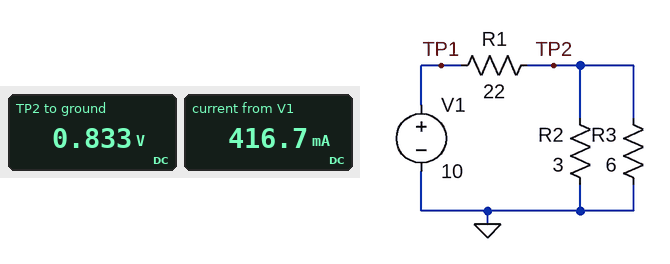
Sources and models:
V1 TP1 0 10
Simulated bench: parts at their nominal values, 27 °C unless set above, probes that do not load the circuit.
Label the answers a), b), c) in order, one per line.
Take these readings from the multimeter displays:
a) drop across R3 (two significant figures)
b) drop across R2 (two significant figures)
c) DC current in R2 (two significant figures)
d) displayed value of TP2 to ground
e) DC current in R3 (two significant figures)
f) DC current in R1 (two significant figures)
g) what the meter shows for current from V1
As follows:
a) 830 mV
b) 830 mV
c) 280 mA
d) 0.833 V
e) 140 mA
f) 420 mA
g) 416.7 mA
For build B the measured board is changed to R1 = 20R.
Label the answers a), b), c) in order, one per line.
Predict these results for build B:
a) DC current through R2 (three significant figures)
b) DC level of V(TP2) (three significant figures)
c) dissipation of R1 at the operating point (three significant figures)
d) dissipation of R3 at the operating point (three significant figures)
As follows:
a) 303 mA
b) 909 mV
c) 4.13 W
d) 138 mW
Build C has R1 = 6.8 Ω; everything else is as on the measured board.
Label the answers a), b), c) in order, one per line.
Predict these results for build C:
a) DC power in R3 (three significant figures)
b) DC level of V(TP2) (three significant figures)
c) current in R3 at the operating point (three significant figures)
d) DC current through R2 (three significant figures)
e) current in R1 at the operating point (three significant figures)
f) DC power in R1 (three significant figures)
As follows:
a) 861 mW
b) 2.27 V
c) 379 mA
d) 758 mA
e) 1.14 A
f) 8.78 W
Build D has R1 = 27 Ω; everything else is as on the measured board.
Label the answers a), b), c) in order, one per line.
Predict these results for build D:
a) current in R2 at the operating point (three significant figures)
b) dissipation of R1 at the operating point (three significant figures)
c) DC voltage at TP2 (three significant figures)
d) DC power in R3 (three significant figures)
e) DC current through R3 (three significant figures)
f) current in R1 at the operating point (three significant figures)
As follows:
a) 230 mA
b) 3.21 W
c) 690 mV
d) 79.3 mW
e) 115 mA
f) 345 mA
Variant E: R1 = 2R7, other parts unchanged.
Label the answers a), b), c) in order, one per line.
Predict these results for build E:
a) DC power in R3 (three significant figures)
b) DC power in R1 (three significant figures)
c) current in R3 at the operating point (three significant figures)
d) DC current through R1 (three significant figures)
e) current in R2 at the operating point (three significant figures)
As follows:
a) 3.02 W
b) 12.2 W
c) 709 mA
d) 2.13 A
e) 1.42 A
